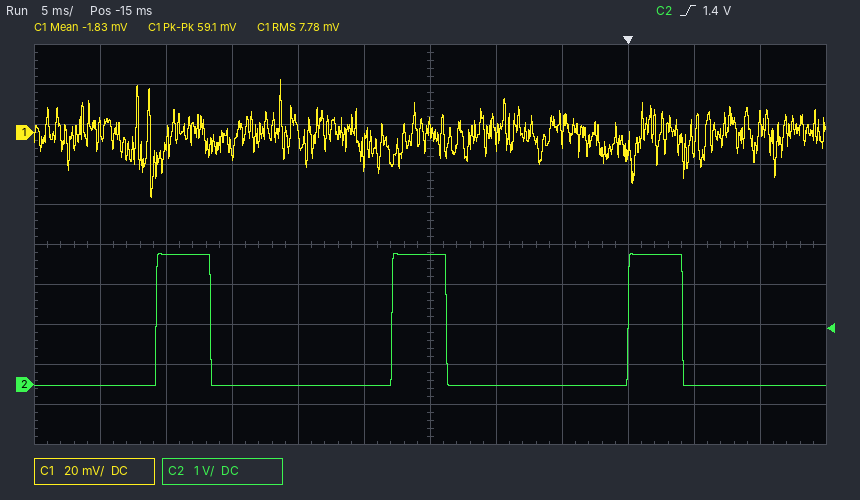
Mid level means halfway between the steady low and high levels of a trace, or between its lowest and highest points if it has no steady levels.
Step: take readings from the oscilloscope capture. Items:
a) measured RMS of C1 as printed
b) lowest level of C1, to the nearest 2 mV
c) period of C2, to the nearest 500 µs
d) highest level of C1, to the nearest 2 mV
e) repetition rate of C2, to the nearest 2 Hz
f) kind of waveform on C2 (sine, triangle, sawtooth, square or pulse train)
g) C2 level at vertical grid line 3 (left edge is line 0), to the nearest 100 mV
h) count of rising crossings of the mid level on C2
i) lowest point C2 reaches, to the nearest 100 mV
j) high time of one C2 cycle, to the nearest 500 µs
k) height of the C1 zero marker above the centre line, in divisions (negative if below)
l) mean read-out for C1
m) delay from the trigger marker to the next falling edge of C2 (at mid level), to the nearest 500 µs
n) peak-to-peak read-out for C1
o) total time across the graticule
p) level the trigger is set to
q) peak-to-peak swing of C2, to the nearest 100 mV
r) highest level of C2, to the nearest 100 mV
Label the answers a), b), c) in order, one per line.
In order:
a) 7.78 mV
b) -32 mV
c) 18.0 ms
d) 26 mV
e) 56 Hz
f) pulse train
g) 0.0 V
h) 3
i) 0.0 V
j) 4.0 ms
k) +2.8 div
l) -1.83 mV
m) 4.0 ms
n) 59.1 mV
o) 60 ms
p) 1.4 V
q) 3.3 V
r) 3.3 V
